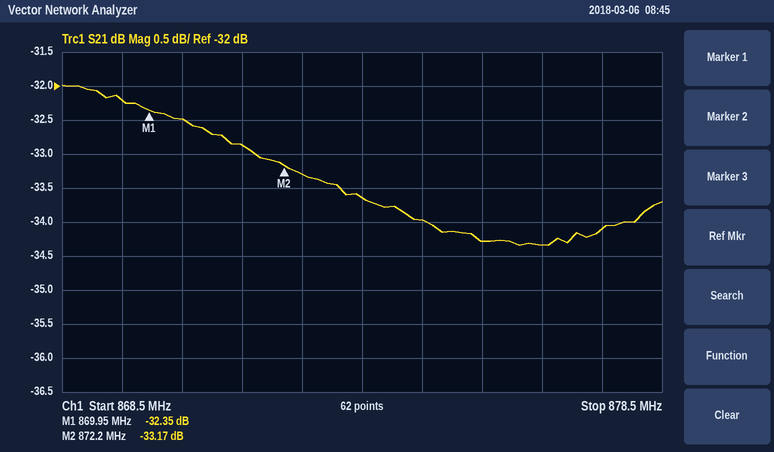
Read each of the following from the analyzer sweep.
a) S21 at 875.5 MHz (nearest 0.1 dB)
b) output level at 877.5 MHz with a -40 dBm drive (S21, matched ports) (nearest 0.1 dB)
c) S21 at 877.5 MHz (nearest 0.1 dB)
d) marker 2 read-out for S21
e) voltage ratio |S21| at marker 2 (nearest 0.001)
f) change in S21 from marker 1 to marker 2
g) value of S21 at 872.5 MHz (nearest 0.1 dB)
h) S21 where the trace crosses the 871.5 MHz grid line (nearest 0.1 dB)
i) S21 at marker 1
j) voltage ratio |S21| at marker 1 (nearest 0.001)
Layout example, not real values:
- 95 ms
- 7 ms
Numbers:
- -34.3 dB
- -74.1 dBm
- -34.1 dB
- -33.17 dB
- 0.022
- -0.82 dB
- -33.3 dB
- -32.9 dB
- -32.35 dB
- 0.024
